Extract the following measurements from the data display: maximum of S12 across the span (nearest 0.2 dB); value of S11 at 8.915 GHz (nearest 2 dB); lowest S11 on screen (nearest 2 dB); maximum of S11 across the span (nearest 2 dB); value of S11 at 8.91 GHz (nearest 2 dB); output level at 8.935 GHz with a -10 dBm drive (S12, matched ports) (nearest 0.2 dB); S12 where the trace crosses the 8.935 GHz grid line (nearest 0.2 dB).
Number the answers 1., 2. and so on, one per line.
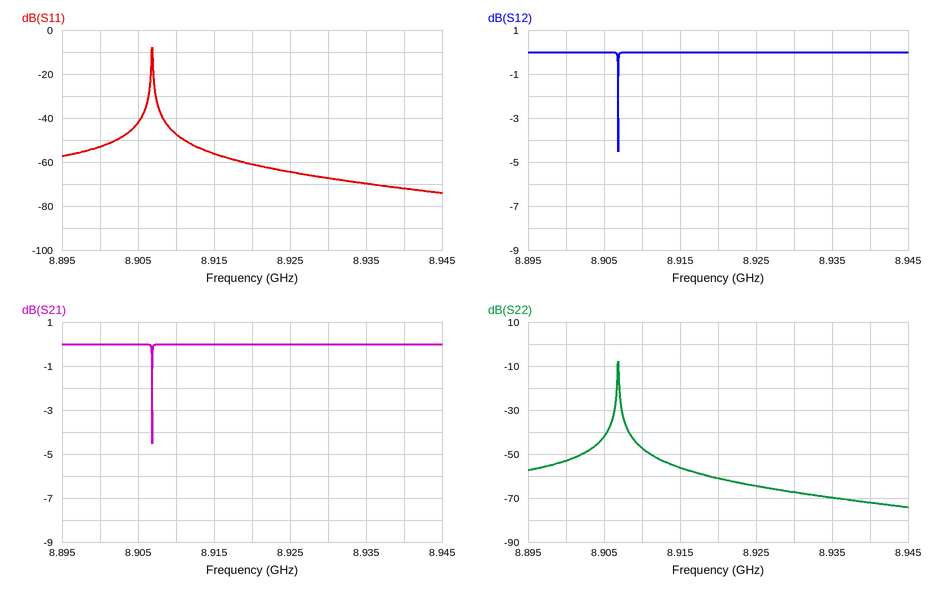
1. 0.0 dB
2. -56 dB
3. -74 dB
4. -8 dB
5. -48 dB
6. -10.0 dBm
7. 0.0 dB
